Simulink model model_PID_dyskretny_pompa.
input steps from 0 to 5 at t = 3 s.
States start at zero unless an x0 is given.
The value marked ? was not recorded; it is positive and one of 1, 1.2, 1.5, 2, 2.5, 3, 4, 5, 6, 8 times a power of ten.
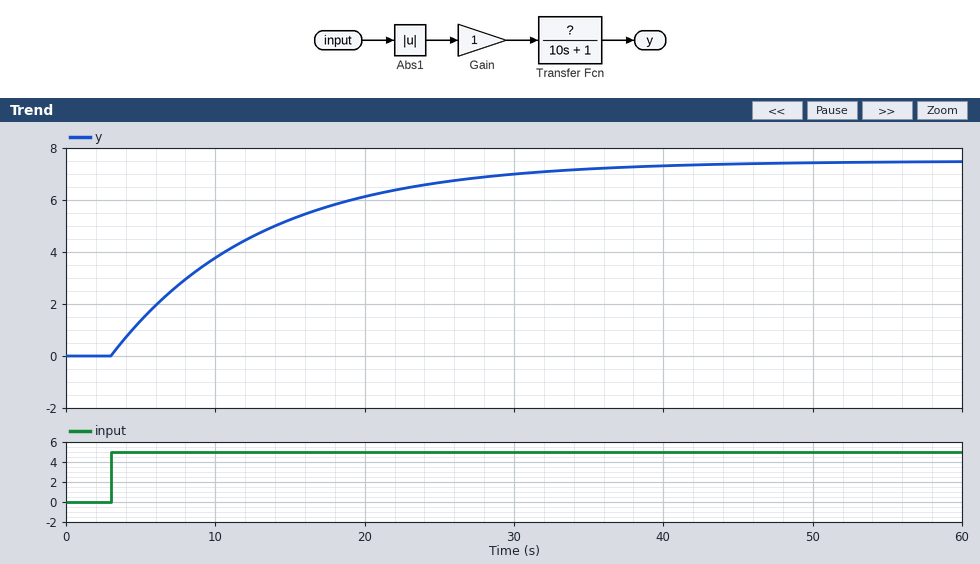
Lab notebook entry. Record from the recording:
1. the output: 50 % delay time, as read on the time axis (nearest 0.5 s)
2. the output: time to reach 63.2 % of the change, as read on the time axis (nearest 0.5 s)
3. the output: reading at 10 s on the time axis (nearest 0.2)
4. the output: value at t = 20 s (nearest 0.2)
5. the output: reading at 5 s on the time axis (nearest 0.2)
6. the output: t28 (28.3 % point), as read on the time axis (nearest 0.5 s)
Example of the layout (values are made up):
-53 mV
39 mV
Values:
10.0 s
13.0 s
3.8
6.2
1.4
6.5 s
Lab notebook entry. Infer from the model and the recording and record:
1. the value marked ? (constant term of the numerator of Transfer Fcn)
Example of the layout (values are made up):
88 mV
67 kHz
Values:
1.5
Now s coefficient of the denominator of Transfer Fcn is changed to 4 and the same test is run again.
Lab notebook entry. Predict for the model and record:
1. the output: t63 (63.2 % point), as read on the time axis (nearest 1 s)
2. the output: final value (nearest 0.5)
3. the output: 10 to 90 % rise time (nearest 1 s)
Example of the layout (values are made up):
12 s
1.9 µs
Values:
7 s
7.5
9 s
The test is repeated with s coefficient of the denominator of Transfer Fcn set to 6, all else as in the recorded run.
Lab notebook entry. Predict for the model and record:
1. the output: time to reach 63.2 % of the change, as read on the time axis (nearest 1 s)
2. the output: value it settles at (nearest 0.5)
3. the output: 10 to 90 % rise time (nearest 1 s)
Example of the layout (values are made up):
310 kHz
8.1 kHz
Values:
9 s
7.5
13 s
